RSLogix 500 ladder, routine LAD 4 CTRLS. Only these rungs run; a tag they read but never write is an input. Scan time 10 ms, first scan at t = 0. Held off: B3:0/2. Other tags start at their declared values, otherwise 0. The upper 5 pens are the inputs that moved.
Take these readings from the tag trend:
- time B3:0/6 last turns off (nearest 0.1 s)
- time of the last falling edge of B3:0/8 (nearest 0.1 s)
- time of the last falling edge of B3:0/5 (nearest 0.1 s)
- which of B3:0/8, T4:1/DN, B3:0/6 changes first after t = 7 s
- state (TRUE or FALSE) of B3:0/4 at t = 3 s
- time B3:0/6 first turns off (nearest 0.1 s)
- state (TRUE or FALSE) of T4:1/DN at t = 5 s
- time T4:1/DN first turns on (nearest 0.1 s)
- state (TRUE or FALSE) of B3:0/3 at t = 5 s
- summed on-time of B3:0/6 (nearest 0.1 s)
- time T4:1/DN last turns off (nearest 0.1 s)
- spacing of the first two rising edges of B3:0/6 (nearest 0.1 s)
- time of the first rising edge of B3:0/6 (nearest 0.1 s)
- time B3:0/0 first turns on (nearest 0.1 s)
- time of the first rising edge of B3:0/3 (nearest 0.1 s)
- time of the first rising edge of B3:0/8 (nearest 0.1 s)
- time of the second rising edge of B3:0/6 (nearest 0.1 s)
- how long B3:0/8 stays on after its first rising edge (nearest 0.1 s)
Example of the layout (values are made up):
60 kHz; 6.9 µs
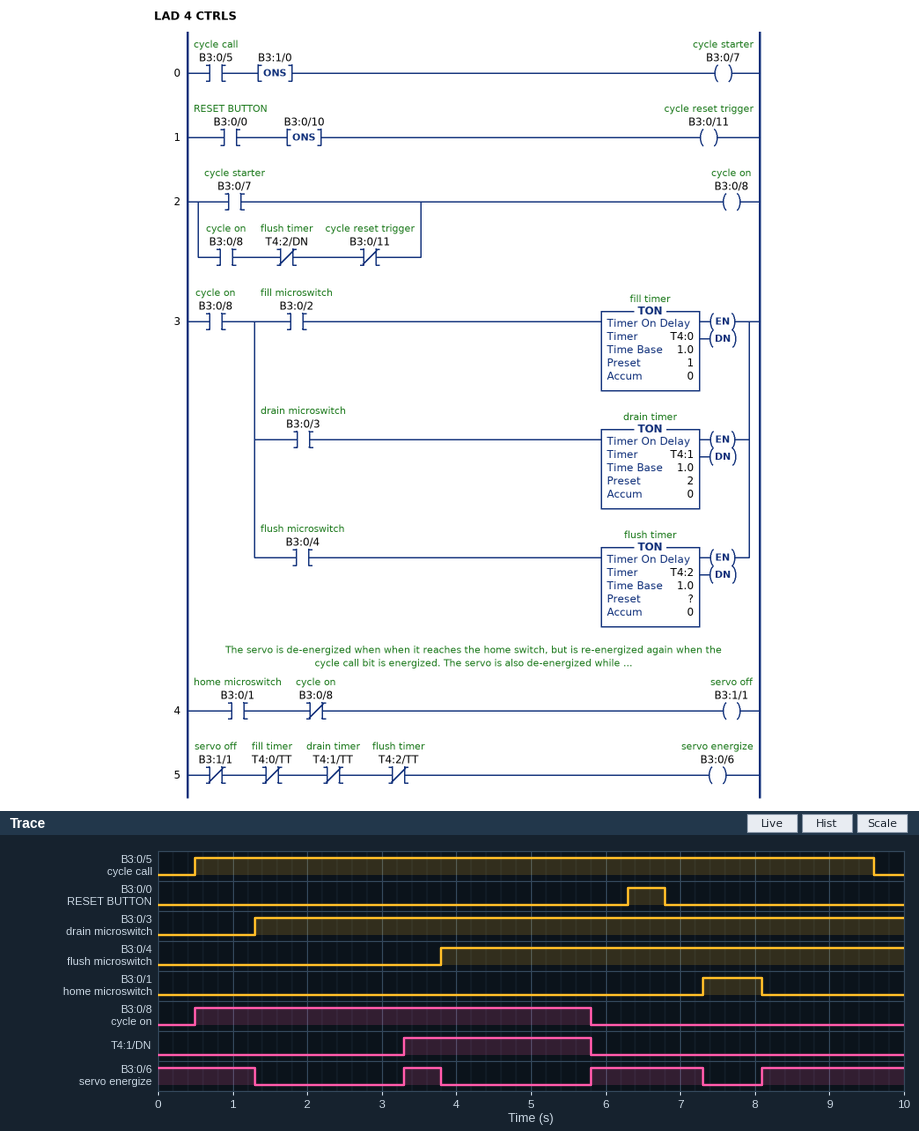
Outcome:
7.3 s; 5.8 s; 9.6 s; B3:0/6; FALSE; 1.3 s; TRUE; 3.3 s; TRUE; 5.2 s; 5.8 s; 2.5 s; 3.3 s; 6.3 s; 1.3 s; 0.5 s; 5.8 s; 5.3 s
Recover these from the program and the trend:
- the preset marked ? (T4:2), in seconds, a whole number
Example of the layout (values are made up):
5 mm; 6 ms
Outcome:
2 s
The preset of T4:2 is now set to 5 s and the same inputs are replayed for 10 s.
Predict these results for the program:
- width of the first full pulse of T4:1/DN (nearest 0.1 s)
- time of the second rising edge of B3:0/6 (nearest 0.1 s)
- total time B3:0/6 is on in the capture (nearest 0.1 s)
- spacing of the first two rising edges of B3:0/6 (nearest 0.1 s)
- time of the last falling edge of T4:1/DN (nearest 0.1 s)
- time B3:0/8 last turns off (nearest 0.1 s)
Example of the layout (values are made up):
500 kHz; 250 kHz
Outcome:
3.0 s; 6.3 s; 4.7 s; 3.0 s; 6.3 s; 6.3 s
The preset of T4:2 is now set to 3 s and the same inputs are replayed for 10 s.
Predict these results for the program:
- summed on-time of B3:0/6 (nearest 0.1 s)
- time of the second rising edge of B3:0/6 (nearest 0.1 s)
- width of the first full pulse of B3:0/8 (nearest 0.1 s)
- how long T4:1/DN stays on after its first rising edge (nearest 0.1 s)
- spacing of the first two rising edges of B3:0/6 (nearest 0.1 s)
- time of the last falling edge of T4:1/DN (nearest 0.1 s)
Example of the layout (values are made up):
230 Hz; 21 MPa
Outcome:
4.7 s; 6.3 s; 5.8 s; 3.0 s; 3.0 s; 6.3 s
